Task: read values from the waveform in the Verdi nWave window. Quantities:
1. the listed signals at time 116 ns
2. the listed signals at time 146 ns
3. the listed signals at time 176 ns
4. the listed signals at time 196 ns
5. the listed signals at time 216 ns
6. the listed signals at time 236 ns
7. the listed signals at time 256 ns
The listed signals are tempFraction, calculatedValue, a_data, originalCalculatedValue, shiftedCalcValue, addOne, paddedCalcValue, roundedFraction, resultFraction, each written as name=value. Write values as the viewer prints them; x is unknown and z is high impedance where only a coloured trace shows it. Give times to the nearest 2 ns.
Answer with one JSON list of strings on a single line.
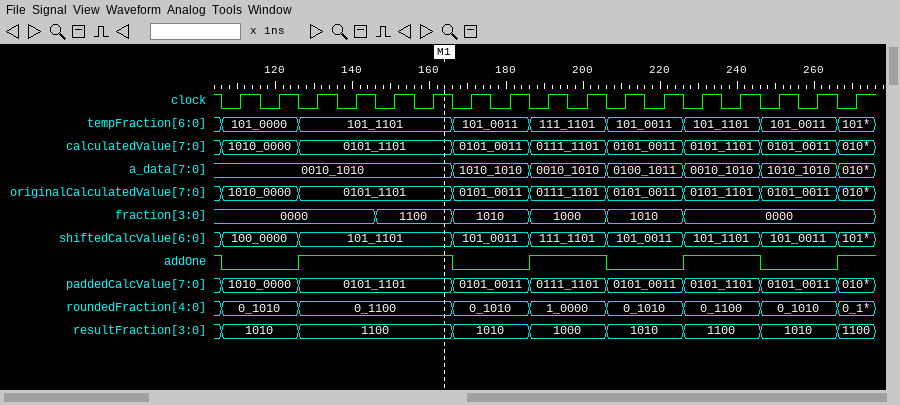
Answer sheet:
["tempFraction=101_0000, calculatedValue=1010_0000, a_data=0010_1010, originalCalculatedValue=1010_0000, shiftedCalcValue=100_0000, addOne=0, paddedCalcValue=1010_0000, roundedFraction=0_1010, resultFraction=1010", "tempFraction=101_1101, calculatedValue=0101_1101, a_data=0010_1010, originalCalculatedValue=0101_1101, shiftedCalcValue=101_1101, addOne=1, paddedCalcValue=0101_1101, roundedFraction=0_1100, resultFraction=1100", "tempFraction=101_0011, calculatedValue=0101_0011, a_data=1010_1010, originalCalculatedValue=0101_0011, shiftedCalcValue=101_0011, addOne=0, paddedCalcValue=0101_0011, roundedFraction=0_1010, resultFraction=1010", "tempFraction=111_1101, calculatedValue=0111_1101, a_data=0010_1010, originalCalculatedValue=0111_1101, shiftedCalcValue=111_1101, addOne=1, paddedCalcValue=0111_1101, roundedFraction=1_0000, resultFraction=1000", "tempFraction=101_0011, calculatedValue=0101_0011, a_data=0100_1011, originalCalculatedValue=0101_0011, shiftedCalcValue=101_0011, addOne=0, paddedCalcValue=0101_0011, roundedFraction=0_1010, resultFraction=1010", "tempFraction=101_1101, calculatedValue=0101_1101, a_data=0010_1010, originalCalculatedValue=0101_1101, shiftedCalcValue=101_1101, addOne=1, paddedCalcValue=0101_1101, roundedFraction=0_1100, resultFraction=1100", "tempFraction=101_0011, calculatedValue=0101_0011, a_data=1010_1010, originalCalculatedValue=0101_0011, shiftedCalcValue=101_0011, addOne=0, paddedCalcValue=0101_0011, roundedFraction=0_1010, resultFraction=1010"]
